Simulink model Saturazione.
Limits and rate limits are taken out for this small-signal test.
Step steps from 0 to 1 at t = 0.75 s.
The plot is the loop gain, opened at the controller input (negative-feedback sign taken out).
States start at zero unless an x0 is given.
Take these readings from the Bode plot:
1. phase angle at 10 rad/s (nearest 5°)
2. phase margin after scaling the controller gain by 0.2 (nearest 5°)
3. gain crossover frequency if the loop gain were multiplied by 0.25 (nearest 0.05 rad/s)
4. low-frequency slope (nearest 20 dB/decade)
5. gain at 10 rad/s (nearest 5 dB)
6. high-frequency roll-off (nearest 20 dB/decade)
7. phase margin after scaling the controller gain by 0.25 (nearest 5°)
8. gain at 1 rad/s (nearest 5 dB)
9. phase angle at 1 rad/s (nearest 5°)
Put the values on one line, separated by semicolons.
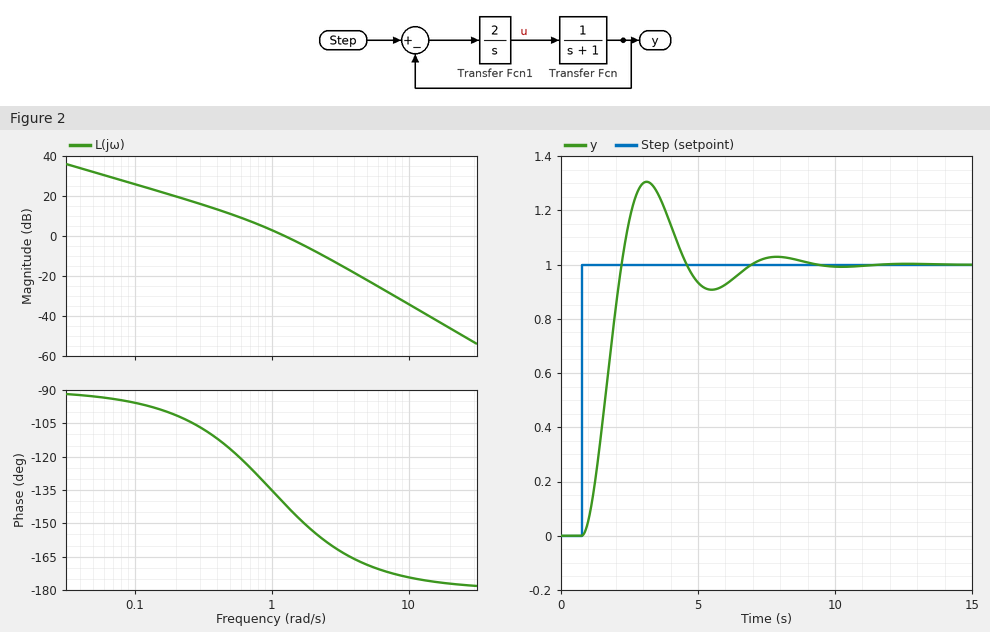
-175°; 70°; 0.45 rad/s; -20 dB/decade; -35 dB; -40 dB/decade; 65°; 5 dB; -135°
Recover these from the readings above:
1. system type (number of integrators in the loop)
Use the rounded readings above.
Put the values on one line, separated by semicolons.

1
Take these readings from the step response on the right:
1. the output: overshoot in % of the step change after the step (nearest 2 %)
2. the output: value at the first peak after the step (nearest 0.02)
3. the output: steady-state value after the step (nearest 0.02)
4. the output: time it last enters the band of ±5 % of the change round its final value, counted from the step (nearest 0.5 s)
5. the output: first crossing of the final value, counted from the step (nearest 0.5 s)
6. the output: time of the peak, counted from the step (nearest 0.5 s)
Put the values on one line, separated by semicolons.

30 %; 1.30; 1.00; 5.5 s; 1.5 s; 2.5 s
